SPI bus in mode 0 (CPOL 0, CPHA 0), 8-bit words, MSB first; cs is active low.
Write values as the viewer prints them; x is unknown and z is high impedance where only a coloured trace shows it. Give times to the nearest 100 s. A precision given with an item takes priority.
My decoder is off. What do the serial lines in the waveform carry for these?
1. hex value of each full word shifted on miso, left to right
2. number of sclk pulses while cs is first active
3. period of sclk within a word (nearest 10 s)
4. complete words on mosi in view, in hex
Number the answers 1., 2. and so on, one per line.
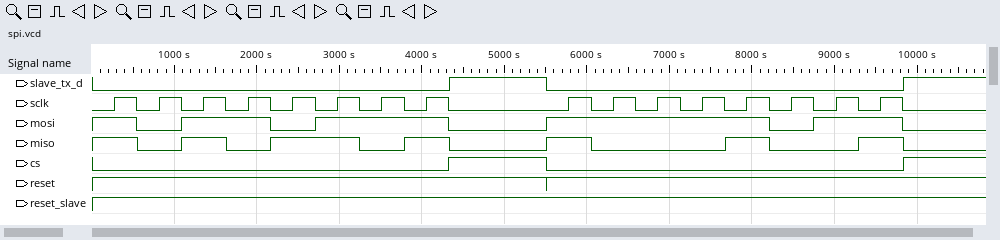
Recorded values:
1. AD, 89
2. 8
3. 540 s
4. B7, FB
